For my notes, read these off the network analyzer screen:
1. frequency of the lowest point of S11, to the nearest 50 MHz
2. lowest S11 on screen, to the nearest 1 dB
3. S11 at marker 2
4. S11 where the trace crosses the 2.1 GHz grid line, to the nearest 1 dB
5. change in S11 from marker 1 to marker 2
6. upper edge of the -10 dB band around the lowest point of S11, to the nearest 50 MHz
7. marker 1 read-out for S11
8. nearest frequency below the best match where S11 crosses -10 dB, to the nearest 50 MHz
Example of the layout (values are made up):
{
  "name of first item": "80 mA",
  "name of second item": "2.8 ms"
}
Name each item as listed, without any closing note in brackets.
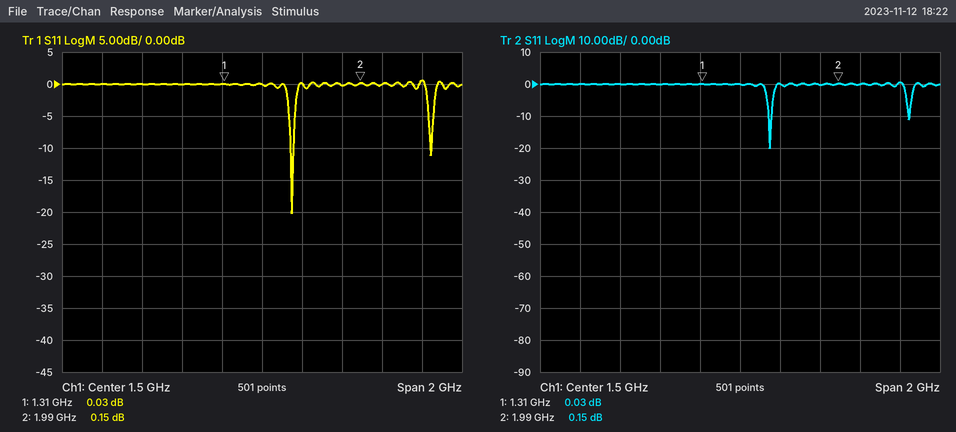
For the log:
{
  "frequency of the lowest point of S11, to the nearest 50 MHz": "1.65 GHz",
  "lowest S11 on screen, to the nearest 1 dB": "-20 dB",
  "S11 at marker 2": "0.15 dB",
  "S11 where the trace crosses the 2.1 GHz grid line, to the nearest 1 dB": "0 dB",
  "change in S11 from marker 1 to marker 2": "0.12 dB",
  "upper edge of the -10 dB band around the lowest point of S11, to the nearest 50 MHz": "1.65 GHz",
  "marker 1 read-out for S11": "0.03 dB",
  "nearest frequency below the best match where S11 crosses -10 dB, to the nearest 50 MHz": "1.65 GHz"
}
